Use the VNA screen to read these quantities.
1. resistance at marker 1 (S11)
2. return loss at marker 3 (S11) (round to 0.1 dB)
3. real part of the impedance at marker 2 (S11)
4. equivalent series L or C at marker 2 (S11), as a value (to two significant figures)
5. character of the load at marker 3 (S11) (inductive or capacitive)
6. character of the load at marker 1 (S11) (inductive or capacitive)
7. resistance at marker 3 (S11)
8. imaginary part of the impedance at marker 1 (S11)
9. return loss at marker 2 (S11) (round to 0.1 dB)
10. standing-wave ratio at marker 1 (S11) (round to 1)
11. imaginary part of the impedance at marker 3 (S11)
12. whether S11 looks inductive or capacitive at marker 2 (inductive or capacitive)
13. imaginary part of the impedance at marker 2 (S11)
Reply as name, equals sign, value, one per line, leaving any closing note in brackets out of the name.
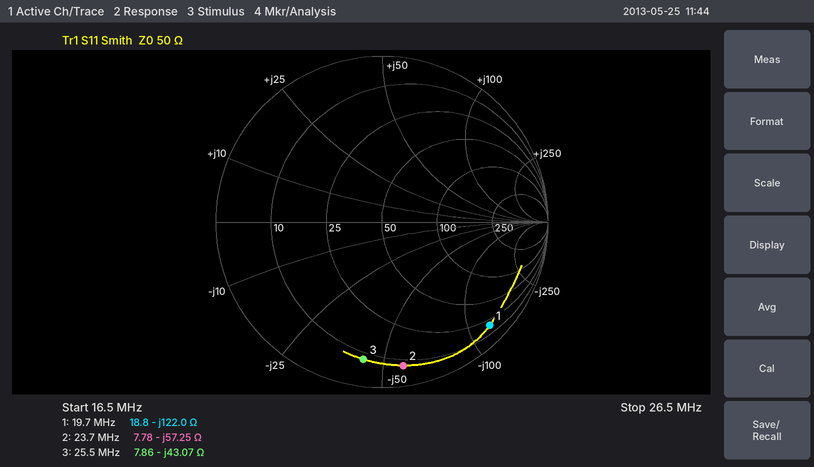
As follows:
resistance at marker 1 = 18.8 Ω
return loss at marker 3 (S11) = 1.6 dB
real part of the impedance at marker 2 = 7.78 Ω
equivalent series L or C at marker 2 (S11), as a value = 120 pF
character of the load at marker 3 (S11) = capacitive
character of the load at marker 1 (S11) = capacitive
resistance at marker 3 = 7.86 Ω
imaginary part of the impedance at marker 1 = -122.0 Ω
return loss at marker 2 (S11) = 1.2 dB
standing-wave ratio at marker 1 (S11) = 19
imaginary part of the impedance at marker 3 = -43.07 Ω
whether S11 looks inductive or capacitive at marker 2 = capacitive
imaginary part of the impedance at marker 2 = -57.25 Ω
